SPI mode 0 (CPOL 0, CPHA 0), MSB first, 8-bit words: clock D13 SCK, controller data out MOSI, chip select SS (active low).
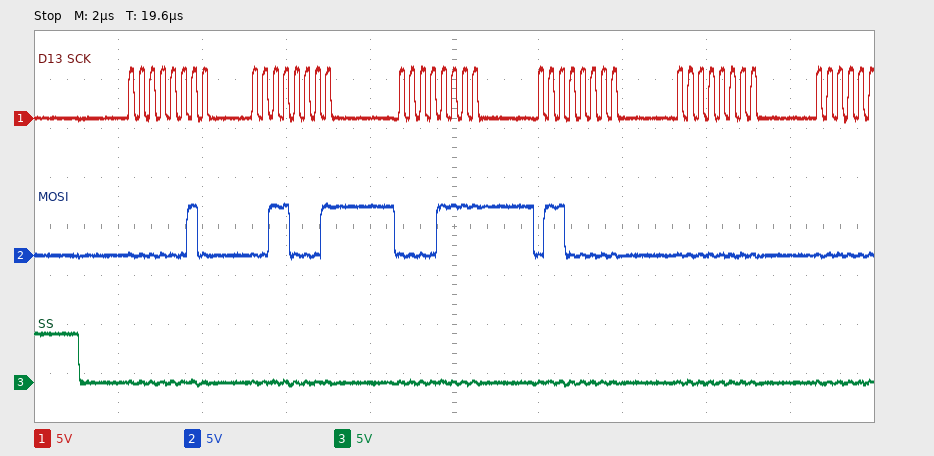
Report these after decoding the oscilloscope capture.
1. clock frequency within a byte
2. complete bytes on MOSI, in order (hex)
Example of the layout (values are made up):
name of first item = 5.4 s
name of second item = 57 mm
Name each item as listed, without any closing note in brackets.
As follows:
clock frequency within a byte = 4 MHz
complete bytes on MOSI, in order = 0x02 0x31 0x0F 0x60 0x00
